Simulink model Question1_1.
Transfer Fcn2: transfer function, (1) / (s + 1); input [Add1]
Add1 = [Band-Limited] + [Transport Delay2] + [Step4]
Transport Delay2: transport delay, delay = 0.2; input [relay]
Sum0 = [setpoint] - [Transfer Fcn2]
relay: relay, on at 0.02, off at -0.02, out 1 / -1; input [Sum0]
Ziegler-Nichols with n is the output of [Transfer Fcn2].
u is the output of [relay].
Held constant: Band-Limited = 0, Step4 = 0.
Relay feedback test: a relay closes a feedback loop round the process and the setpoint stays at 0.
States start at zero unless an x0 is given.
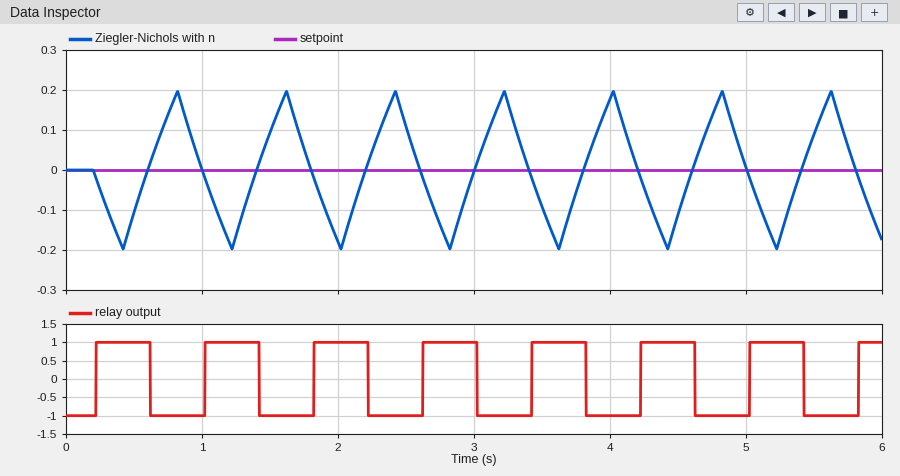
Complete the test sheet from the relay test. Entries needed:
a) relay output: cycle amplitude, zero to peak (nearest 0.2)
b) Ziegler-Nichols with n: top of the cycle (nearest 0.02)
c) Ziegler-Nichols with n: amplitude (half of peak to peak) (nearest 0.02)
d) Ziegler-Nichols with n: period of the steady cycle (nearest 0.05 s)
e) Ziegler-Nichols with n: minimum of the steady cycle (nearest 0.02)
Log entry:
1.0
0.20
0.20
0.80 s
-0.20
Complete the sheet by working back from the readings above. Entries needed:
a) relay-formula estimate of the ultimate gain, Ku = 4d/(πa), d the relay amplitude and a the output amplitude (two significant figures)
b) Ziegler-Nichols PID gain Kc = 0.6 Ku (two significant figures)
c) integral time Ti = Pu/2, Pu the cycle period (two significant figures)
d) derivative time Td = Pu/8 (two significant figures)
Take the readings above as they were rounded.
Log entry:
6.4
3.8
0.40 s
0.10 s
